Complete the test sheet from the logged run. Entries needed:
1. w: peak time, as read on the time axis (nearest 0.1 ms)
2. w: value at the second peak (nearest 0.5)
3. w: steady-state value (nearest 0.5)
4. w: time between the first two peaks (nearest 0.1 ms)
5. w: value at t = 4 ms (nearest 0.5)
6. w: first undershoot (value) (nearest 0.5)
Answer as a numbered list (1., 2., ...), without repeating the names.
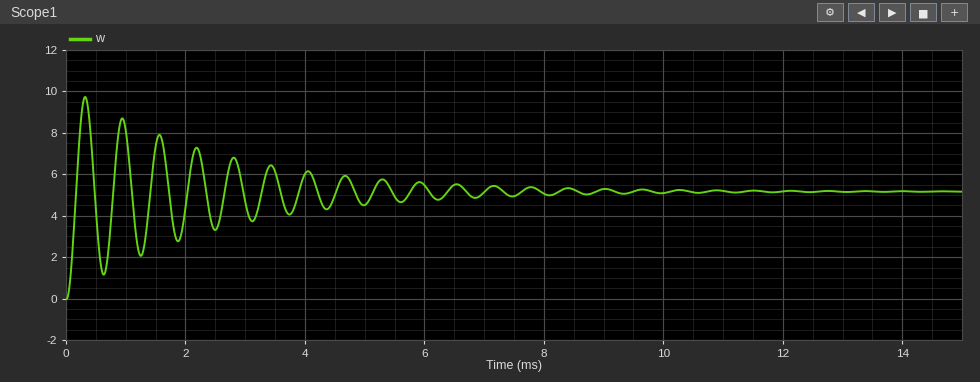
1. 0.3 ms
2. 8.5
3. 5.0
4. 0.6 ms
5. 6.0
6. 1.0
